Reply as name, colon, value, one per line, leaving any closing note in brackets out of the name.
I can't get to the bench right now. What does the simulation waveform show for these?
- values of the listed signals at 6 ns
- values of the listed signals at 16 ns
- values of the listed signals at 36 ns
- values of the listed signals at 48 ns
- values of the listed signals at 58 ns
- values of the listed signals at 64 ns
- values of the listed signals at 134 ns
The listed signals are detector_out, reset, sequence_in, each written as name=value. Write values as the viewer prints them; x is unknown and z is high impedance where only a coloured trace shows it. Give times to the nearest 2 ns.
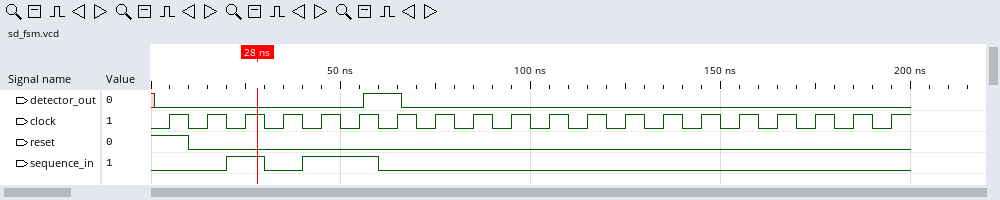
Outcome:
values of the listed signals at 6 ns: detector_out=0, reset=1, sequence_in=0
values of the listed signals at 16 ns: detector_out=0, reset=0, sequence_in=0
values of the listed signals at 36 ns: detector_out=0, reset=0, sequence_in=0
values of the listed signals at 48 ns: detector_out=0, reset=0, sequence_in=1
values of the listed signals at 58 ns: detector_out=1, reset=0, sequence_in=1
values of the listed signals at 64 ns: detector_out=1, reset=0, sequence_in=0
values of the listed signals at 134 ns: detector_out=0, reset=0, sequence_in=0
